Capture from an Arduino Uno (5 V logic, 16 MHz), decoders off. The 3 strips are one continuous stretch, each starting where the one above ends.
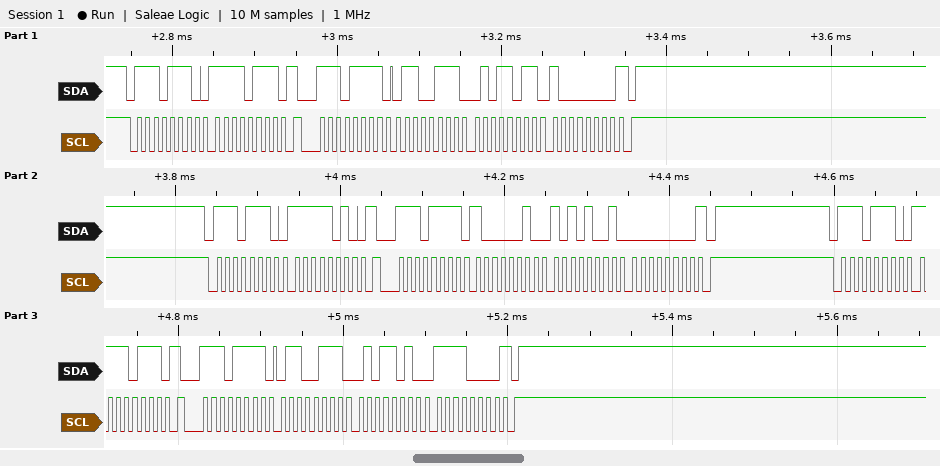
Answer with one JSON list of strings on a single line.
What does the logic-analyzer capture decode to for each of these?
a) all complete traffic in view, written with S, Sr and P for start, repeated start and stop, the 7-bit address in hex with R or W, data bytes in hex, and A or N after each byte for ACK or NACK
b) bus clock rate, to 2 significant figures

["S 77W A F7 A Sr 77R A 67 A 5B A 80 N P S 77W A FA A Sr 77R A 82 A A9 A 00 N P S 77W A F7 A Sr 77R A 67 A 5A A F0 N P", "100 kHz"]
